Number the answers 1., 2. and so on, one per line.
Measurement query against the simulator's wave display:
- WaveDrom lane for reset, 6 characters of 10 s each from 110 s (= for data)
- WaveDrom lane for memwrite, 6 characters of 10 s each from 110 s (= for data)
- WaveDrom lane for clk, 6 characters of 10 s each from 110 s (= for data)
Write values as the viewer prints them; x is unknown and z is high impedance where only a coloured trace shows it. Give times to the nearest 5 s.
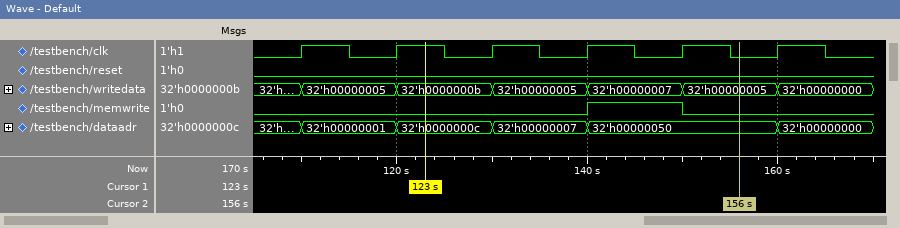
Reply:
1. {name: 'reset', wave: '0.....'}
2. {name: 'memwrite', wave: '0..10.'}
3. {name: 'clk', wave: 'p.....'}
